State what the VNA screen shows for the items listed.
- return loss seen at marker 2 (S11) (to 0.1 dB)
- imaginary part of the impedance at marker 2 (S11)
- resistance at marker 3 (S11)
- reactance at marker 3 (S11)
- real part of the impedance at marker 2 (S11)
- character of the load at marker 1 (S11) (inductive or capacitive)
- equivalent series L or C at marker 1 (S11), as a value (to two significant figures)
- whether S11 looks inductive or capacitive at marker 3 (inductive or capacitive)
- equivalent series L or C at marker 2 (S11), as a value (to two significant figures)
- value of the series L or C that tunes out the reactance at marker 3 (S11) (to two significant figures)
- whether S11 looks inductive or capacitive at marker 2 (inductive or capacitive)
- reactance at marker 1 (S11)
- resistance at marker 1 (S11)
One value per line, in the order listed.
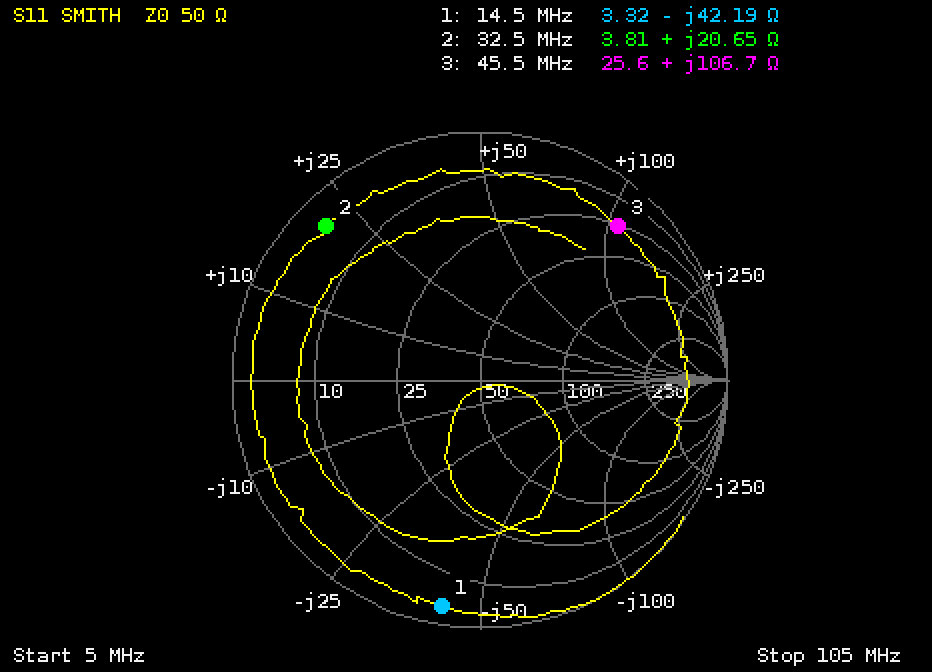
1.1 dB
+20.65 Ω
25.6 Ω
+106.7 Ω
3.81 Ω
capacitive
260 pF
inductive
100 nH
33 pF
inductive
-42.19 Ω
3.32 Ω
